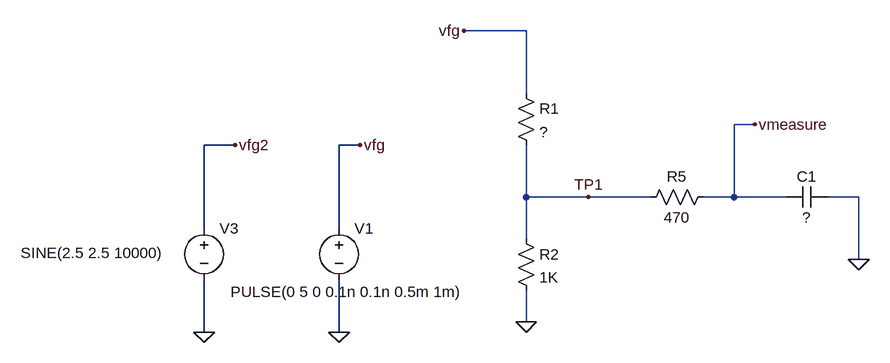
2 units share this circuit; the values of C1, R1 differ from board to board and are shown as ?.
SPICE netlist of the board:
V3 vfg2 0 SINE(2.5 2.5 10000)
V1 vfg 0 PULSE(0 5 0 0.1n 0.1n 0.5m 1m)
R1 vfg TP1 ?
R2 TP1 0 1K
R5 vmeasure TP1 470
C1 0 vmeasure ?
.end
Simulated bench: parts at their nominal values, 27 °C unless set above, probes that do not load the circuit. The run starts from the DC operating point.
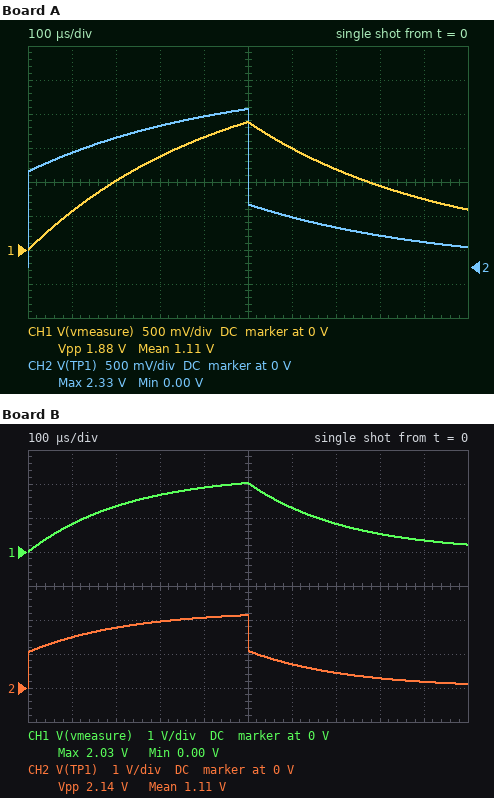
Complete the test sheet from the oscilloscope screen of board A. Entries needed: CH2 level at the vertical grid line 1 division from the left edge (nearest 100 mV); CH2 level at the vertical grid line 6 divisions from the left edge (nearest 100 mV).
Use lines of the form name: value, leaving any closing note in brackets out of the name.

CH2 level at the vertical grid line 1 division from the left edge: 1.7 V
CH2 level at the vertical grid line 6 divisions from the left edge: 700 mV
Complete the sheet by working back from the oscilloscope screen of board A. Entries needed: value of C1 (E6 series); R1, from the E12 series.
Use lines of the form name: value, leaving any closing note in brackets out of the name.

value of C1: 470 nF
R1, from the E12 series: 820 Ω
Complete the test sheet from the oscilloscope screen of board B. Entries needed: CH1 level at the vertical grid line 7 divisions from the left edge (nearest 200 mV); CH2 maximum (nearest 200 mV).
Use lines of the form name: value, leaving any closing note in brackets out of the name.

CH1 level at the vertical grid line 7 divisions from the left edge: 800 mV
CH2 maximum: 2.2 V
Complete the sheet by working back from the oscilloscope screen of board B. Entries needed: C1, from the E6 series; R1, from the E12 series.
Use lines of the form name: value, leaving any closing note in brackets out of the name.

C1, from the E6 series: 220 nF
R1, from the E12 series: 1.2 kΩ
